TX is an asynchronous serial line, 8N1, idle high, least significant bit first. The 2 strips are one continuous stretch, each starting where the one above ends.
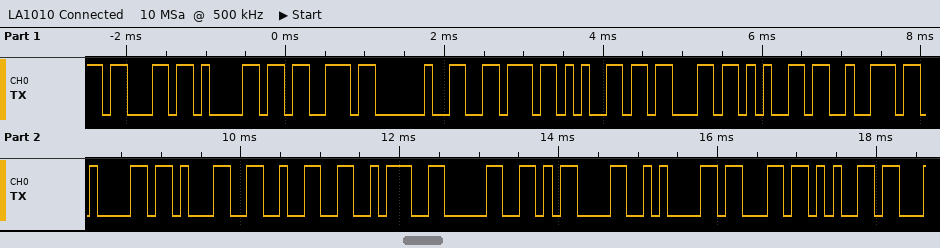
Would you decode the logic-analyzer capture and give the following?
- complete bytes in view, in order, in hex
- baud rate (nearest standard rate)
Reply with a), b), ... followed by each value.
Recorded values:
a) 63 61 73 20 76 65 63 65 72 61 31 32 3A 30 0D 0A 63 65
b) 9600 baud
